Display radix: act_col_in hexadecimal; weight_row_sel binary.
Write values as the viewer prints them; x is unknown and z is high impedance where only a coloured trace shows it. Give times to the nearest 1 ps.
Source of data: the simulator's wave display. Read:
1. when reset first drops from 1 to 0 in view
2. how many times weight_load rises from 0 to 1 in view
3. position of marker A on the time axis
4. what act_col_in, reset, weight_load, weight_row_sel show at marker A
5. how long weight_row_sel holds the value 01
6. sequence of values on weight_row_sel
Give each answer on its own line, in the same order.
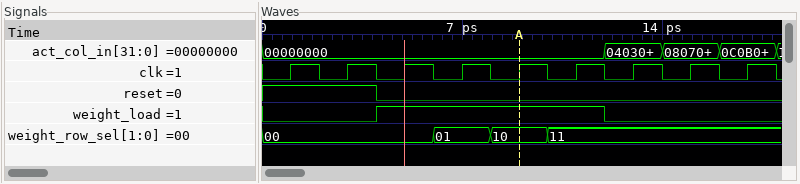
4 ps
1
9 ps
act_col_in=00000000, reset=0, weight_load=1, weight_row_sel=10
2 ps
00, 01, 10, 11
